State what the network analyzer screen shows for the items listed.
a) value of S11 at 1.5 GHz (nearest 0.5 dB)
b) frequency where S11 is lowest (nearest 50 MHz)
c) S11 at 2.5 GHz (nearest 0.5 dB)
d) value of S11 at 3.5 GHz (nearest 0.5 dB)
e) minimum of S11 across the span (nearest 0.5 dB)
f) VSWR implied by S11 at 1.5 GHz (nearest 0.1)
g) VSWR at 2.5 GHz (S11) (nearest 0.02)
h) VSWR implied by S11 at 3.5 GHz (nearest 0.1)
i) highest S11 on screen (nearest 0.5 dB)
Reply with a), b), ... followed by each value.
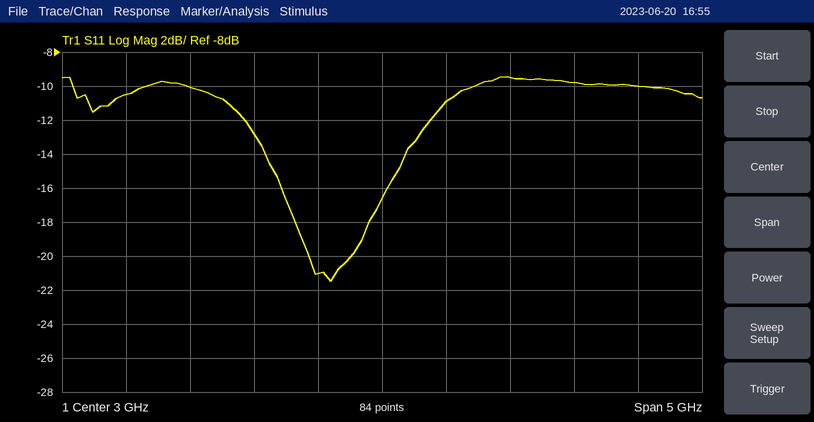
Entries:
a) -10.0 dB
b) 2.60 GHz
c) -21.0 dB
d) -11.0 dB
e) -21.5 dB
f) 1.9
g) 1.20
h) 1.8
i) -9.5 dB
